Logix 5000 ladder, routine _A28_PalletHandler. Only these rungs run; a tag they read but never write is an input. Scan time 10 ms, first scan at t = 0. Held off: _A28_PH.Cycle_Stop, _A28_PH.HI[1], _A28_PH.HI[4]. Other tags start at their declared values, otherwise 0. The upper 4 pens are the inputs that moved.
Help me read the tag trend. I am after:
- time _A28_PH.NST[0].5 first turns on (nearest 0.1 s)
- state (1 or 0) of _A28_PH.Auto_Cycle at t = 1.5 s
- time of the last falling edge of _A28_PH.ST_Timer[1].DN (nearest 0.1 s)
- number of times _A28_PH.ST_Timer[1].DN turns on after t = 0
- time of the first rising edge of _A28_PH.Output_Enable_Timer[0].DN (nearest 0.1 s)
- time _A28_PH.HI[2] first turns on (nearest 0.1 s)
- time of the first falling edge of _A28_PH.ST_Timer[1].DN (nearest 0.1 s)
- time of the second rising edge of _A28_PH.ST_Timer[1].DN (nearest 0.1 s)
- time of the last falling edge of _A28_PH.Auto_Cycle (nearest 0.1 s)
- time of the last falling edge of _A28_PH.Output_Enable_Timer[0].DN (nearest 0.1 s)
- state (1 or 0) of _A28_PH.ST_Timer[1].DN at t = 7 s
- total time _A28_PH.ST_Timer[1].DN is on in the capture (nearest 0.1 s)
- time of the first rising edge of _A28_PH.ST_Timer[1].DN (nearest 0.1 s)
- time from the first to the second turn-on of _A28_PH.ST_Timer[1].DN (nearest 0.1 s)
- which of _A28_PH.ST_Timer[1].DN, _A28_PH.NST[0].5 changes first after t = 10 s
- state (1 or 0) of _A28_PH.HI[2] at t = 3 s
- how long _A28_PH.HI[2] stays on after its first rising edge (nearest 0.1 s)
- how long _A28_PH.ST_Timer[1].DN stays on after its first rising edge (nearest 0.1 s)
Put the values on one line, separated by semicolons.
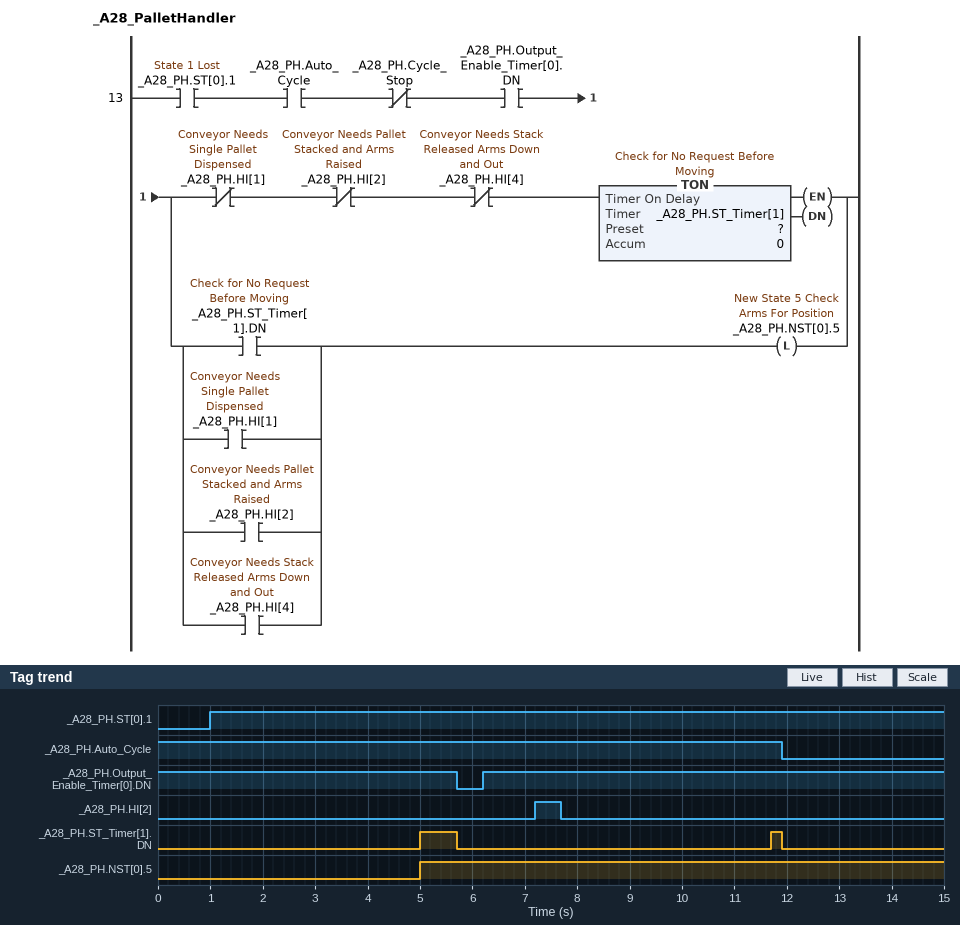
5.0 s; 1; 11.9 s; 2; 6.2 s; 7.2 s; 5.7 s; 11.7 s; 11.9 s; 5.7 s; 0; 0.9 s; 5.0 s; 6.7 s; _A28_PH.ST_Timer[1].DN; 0; 0.5 s; 0.7 s
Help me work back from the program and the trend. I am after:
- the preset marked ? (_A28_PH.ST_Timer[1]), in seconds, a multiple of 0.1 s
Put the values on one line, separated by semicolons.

4.0 s
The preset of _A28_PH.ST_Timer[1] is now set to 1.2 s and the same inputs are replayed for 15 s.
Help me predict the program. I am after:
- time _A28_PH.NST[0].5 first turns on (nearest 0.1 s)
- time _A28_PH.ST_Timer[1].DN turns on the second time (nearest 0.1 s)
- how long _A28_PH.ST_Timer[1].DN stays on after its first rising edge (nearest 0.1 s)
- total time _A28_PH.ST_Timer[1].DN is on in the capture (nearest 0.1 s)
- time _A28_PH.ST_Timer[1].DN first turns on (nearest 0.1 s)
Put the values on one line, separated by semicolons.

2.2 s; 8.9 s; 3.5 s; 6.5 s; 2.2 s
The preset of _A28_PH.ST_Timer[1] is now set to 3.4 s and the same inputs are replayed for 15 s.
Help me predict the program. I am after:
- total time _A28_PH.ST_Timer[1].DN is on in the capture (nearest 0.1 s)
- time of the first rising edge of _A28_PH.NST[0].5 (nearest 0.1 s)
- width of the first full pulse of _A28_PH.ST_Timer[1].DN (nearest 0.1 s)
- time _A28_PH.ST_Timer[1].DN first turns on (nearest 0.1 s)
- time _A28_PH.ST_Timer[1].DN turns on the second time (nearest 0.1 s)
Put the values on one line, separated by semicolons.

2.1 s; 4.4 s; 1.3 s; 4.4 s; 11.1 s
